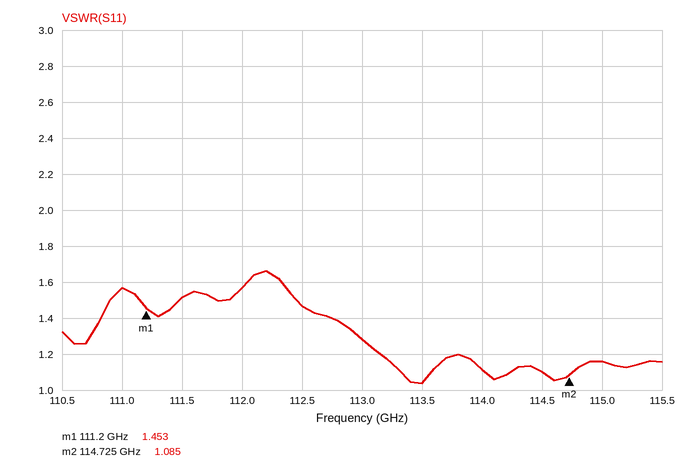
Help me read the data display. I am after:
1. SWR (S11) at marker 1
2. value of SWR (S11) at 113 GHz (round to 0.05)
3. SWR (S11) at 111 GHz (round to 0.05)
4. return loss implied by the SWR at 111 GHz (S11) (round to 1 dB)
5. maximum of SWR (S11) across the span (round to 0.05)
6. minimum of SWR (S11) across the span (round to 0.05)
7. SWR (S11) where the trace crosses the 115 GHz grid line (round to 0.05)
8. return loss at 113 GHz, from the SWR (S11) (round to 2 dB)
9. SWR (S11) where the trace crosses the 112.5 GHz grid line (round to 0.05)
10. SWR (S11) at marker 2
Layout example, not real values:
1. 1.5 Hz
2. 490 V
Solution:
1. 1.453
2. 1.30
3. 1.55
4. 13 dB
5. 1.65
6. 1.05
7. 1.15
8. 18 dB
9. 1.45
10. 1.085
